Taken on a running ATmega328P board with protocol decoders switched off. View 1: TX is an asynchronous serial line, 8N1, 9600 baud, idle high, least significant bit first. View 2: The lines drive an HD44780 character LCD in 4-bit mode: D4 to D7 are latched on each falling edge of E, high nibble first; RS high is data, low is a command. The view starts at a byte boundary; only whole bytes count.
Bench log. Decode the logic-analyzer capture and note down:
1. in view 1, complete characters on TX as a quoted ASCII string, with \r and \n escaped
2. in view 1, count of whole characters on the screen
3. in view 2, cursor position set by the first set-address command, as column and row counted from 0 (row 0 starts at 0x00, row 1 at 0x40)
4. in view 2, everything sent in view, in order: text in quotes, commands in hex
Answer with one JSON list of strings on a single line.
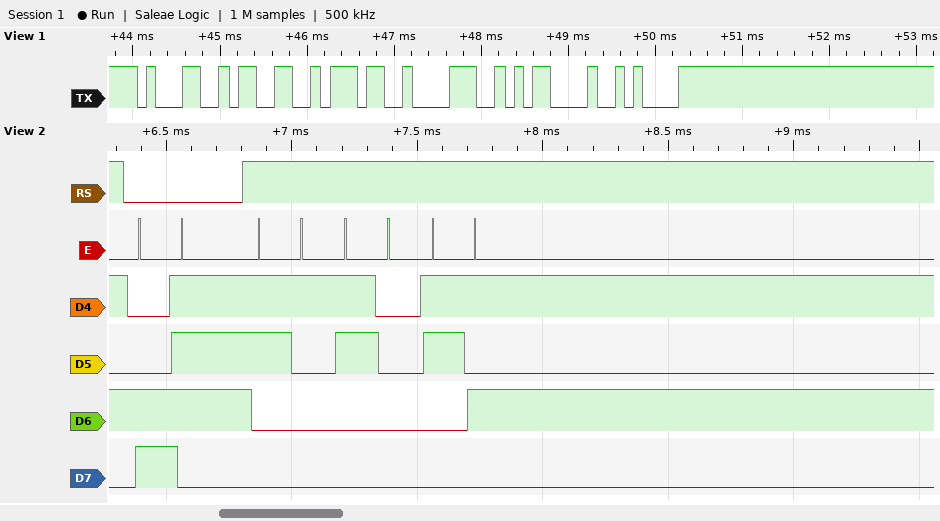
["\"1378\\r\\n\"", "6", "column 7, row 1", "0xC7 \"105\""]
